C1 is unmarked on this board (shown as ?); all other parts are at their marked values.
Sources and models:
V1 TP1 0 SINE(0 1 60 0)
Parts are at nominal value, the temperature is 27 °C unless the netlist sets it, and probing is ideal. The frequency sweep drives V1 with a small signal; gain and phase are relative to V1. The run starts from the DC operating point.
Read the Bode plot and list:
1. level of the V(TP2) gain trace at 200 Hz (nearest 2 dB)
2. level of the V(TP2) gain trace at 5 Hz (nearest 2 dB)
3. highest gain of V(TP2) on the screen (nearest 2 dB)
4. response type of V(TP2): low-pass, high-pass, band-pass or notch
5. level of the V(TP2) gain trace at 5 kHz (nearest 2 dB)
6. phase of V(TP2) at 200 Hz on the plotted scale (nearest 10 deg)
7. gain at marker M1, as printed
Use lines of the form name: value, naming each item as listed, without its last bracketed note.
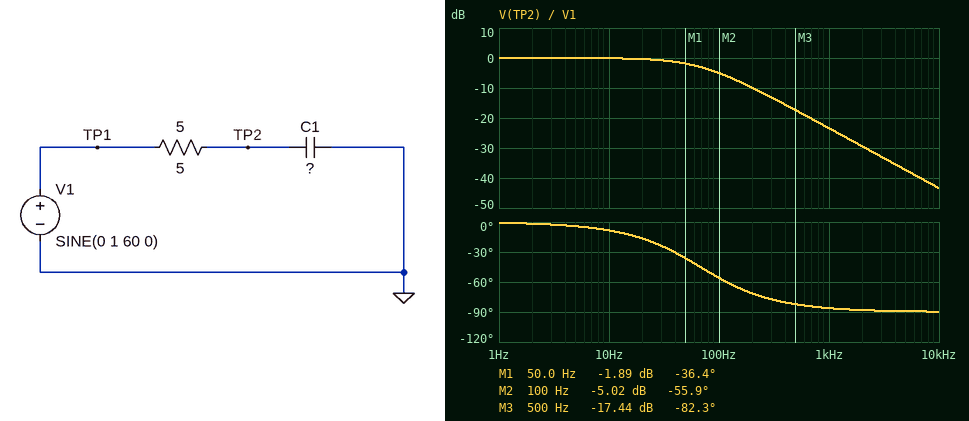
level of the V(TP2) gain trace at 200 Hz: -10 dB
level of the V(TP2) gain trace at 5 Hz: 0 dB
highest gain of V(TP2) on the screen: 0 dB
response type of V(TP2): low-pass, high-pass, band-pass or notch: low-pass
level of the V(TP2) gain trace at 5 kHz: -38 dB
phase of V(TP2) at 200 Hz on the plotted scale: -70 deg
gain at marker M1, as printed: -1.89 dB
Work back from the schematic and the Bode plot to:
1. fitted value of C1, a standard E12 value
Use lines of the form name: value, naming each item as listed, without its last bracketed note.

fitted value of C1, a standard E12 value: 470 µF
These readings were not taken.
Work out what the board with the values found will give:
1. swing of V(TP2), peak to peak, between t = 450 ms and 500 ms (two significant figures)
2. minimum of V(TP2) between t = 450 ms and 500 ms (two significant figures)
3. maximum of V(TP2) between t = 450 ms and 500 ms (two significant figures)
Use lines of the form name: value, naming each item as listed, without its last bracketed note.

swing of V(TP2), peak to peak, between t = 450 ms and 500 ms: 1.5 V
minimum of V(TP2) between t = 450 ms and 500 ms: -750 mV
maximum of V(TP2) between t = 450 ms and 500 ms: 750 mV
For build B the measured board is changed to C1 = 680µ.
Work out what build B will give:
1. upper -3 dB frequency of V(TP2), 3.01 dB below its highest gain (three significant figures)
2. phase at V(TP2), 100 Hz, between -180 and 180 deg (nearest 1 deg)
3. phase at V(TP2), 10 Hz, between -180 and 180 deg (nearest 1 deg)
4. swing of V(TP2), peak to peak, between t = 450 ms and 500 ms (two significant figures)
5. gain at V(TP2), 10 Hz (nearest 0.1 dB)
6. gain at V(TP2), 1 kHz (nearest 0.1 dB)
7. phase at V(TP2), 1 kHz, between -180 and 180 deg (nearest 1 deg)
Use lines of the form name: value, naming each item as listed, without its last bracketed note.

upper -3 dB frequency of V(TP2), 3.01 dB below its highest gain: 46.8 Hz
phase at V(TP2), 100 Hz, between -180 and 180 deg: -65 deg
phase at V(TP2), 10 Hz, between -180 and 180 deg: -12 deg
swing of V(TP2), peak to peak, between t = 450 ms and 500 ms: 1.2 V
gain at V(TP2), 10 Hz: -0.2 dB
gain at V(TP2), 1 kHz: -26.6 dB
phase at V(TP2), 1 kHz, between -180 and 180 deg: -87 deg
